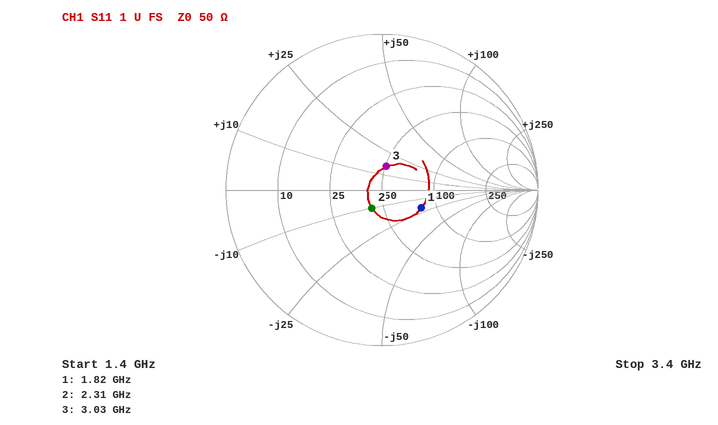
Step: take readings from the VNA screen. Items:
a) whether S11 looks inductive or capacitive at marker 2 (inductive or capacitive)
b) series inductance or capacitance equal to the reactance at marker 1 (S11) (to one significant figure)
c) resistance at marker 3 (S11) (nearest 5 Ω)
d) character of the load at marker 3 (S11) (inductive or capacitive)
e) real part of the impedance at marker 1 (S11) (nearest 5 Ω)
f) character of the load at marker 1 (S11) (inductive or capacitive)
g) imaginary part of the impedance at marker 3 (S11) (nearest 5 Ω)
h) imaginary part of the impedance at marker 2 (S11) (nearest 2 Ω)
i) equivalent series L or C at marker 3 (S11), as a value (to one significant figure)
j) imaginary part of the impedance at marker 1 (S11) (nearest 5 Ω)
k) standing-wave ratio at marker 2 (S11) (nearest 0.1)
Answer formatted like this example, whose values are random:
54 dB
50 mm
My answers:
capacitive
4 pF
50 Ω
inductive
80 Ω
capacitive
+15 Ω
-10 Ω
800 pH
-20 Ω
1.3
